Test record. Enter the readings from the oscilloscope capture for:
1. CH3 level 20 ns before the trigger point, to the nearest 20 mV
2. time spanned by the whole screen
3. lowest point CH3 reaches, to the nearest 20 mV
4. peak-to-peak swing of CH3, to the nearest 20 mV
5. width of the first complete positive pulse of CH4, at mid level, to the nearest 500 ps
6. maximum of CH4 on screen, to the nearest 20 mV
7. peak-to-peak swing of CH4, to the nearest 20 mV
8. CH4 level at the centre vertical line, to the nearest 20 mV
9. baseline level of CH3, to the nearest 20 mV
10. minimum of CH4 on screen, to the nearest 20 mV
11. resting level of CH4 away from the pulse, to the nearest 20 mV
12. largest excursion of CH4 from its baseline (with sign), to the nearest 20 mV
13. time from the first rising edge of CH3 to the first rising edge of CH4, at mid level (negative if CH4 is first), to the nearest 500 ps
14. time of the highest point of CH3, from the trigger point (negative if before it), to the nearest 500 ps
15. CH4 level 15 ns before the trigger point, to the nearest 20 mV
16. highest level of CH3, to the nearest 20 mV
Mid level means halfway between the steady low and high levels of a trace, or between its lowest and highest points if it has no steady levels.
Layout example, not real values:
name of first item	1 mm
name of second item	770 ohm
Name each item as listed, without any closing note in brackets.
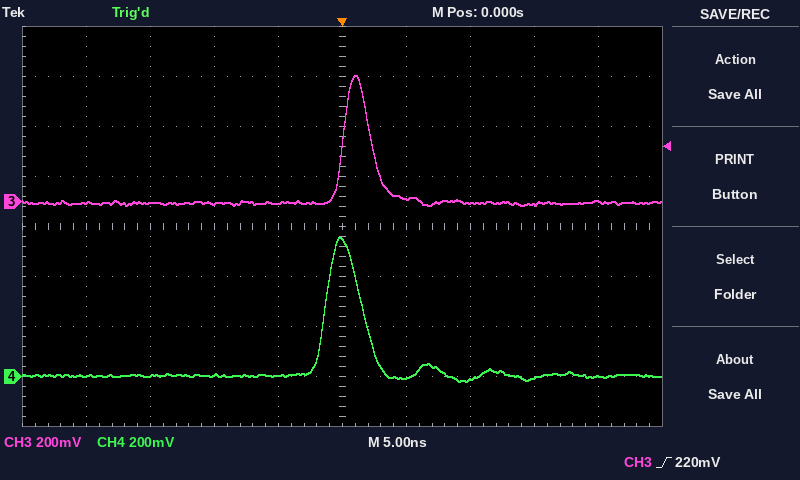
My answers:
CH3 level 20 ns before the trigger point, to the nearest 20 mV	0 mV
time spanned by the whole screen	50 ns
lowest point CH3 reaches, to the nearest 20 mV	-20 mV
peak-to-peak swing of CH3, to the nearest 20 mV	520 mV
width of the first complete positive pulse of CH4, at mid level, to the nearest 500 ps	3.0 ns
maximum of CH4 on screen, to the nearest 20 mV	560 mV
peak-to-peak swing of CH4, to the nearest 20 mV	580 mV
CH4 level at the centre vertical line, to the nearest 20 mV	540 mV
baseline level of CH3, to the nearest 20 mV	0 mV
minimum of CH4 on screen, to the nearest 20 mV	-20 mV
resting level of CH4 away from the pulse, to the nearest 20 mV	0 mV
largest excursion of CH4 from its baseline (with sign), to the nearest 20 mV	+560 mV
time from the first rising edge of CH3 to the first rising edge of CH4, at mid level (negative if CH4 is first), to the nearest 500 ps	-1.5 ns
time of the highest point of CH3, from the trigger point (negative if before it), to the nearest 500 ps	+1.0 ns
CH4 level 15 ns before the trigger point, to the nearest 20 mV	0 mV
highest level of CH3, to the nearest 20 mV	500 mV
